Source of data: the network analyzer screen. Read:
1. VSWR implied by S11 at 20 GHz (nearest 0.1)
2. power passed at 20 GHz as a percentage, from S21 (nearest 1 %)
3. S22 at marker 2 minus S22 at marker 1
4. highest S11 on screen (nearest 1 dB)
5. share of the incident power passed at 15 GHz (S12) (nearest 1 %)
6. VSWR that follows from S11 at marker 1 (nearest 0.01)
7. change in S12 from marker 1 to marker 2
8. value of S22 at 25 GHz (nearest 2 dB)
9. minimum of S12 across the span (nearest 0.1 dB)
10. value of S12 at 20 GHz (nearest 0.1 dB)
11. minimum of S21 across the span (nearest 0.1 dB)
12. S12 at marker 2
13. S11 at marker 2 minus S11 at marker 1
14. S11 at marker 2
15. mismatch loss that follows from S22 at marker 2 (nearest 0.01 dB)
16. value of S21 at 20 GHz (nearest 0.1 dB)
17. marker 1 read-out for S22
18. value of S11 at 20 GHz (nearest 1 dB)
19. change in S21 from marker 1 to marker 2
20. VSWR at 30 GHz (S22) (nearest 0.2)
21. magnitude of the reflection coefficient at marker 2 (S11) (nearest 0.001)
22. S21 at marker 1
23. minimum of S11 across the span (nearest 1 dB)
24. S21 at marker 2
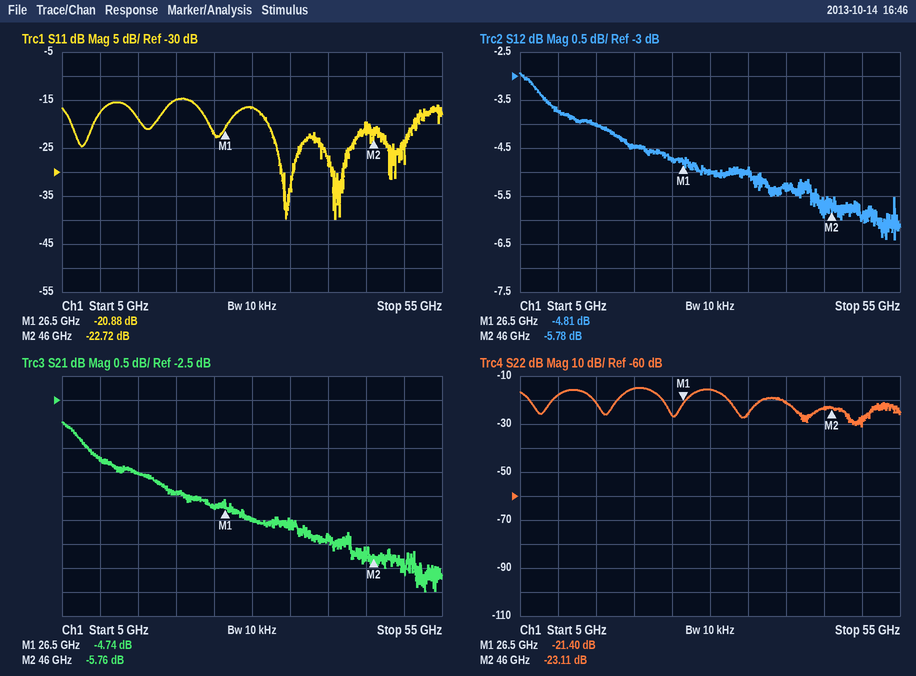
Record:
1.4
36 %
-1.71 dB
-15 dB
40 %
1.20
-0.97 dB
-26 dB
-6.4 dB
-4.5 dB
-6.5 dB
-5.78 dB
-1.84 dB
-22.72 dB
0.02 dB
-4.4 dB
-21.40 dB
-15 dB
-1.02 dB
1.4
0.073
-4.74 dB
-40 dB
-5.76 dB
